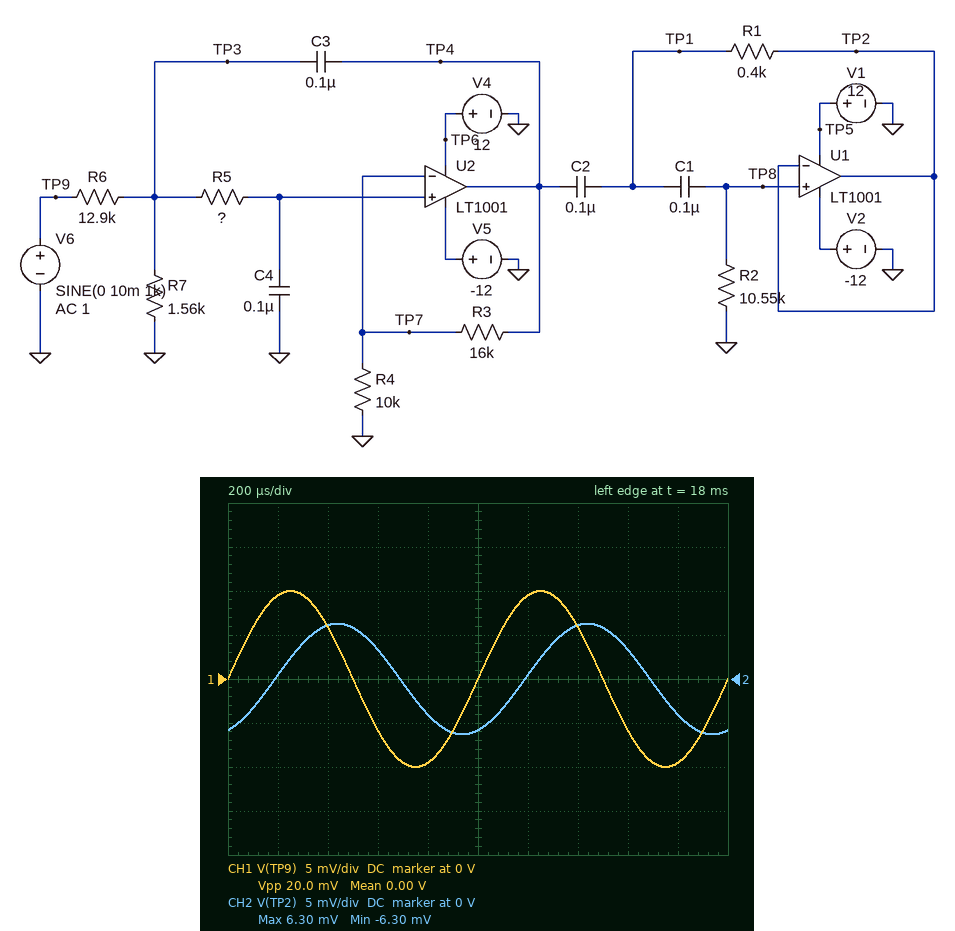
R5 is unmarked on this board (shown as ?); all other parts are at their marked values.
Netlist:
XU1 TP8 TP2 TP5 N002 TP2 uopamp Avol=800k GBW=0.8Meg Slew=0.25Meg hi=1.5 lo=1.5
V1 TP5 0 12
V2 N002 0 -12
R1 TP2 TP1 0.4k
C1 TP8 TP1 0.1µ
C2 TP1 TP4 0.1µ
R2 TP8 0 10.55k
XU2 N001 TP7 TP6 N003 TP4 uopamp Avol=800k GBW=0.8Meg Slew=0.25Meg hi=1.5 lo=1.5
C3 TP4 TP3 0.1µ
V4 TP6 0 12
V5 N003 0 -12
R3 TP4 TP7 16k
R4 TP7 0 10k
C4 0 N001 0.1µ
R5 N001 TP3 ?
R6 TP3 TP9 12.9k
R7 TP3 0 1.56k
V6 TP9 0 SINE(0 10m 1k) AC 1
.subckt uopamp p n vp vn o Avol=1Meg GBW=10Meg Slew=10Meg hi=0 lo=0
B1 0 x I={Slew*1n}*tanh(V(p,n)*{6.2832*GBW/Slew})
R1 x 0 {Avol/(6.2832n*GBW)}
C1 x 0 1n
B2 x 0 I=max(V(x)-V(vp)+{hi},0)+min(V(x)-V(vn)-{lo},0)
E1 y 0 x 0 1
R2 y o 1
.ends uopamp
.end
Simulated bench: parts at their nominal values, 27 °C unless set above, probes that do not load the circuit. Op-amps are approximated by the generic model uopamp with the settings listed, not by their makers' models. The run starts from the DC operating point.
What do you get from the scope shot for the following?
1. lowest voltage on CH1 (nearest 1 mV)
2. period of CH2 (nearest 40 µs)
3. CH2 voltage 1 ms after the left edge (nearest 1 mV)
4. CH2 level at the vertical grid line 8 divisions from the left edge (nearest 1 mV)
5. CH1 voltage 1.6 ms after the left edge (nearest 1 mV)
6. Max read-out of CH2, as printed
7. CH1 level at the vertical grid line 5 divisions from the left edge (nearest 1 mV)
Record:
-10 mV
1.00 ms
-6 mV
3 mV
-6 mV
6.30 mV
0 V
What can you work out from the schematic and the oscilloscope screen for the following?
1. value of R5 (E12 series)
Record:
2.2 kΩ
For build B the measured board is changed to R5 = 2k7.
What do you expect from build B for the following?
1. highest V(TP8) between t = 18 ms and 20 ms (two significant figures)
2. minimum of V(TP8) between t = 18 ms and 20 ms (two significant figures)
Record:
4.4 mV
-4.4 mV
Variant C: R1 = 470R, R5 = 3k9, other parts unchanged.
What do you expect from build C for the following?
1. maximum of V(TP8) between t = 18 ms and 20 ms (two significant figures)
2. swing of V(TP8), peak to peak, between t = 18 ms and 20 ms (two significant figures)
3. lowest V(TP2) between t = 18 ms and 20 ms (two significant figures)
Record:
2.2 mV
4.3 mV
-2.2 mV
